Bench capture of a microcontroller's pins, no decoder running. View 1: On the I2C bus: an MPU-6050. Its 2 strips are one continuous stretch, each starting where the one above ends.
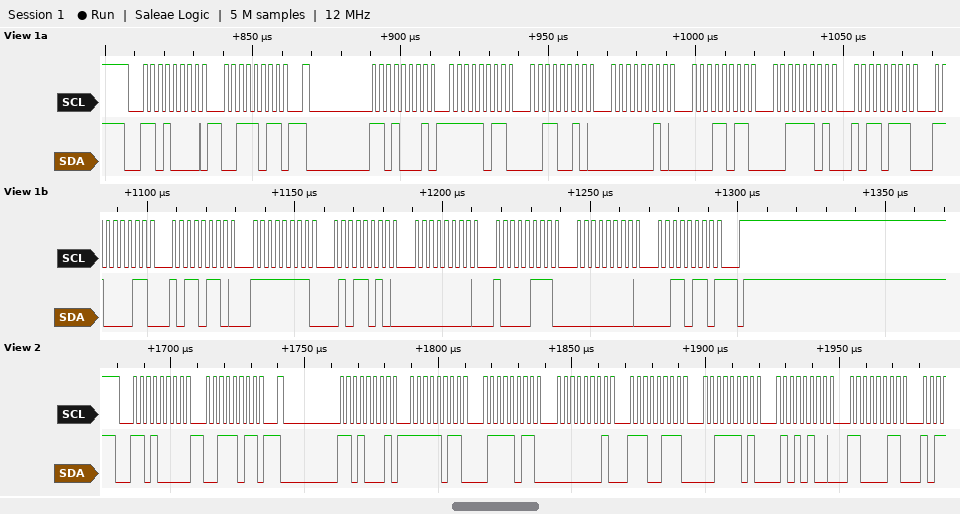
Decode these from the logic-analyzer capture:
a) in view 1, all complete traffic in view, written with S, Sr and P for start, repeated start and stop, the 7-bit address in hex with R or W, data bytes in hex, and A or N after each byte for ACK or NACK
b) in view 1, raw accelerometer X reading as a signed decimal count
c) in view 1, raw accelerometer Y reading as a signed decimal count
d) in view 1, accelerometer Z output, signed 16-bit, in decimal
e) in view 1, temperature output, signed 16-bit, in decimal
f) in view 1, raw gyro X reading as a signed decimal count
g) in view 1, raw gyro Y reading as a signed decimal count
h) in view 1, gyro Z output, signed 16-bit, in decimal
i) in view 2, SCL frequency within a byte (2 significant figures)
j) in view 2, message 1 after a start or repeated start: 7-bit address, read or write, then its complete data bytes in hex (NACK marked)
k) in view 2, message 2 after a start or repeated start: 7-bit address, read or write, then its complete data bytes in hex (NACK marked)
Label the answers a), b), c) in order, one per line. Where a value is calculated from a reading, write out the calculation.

a) S 68W A 3B A Sr 68R A FB A 32 A 02 A 1B A 3D A B7 A C3 A B6 A FF A 5A A 00 A 87 A 00 A 36 N P
b) 0xFB32 = -1230
c) 0x021B = 539
d) 0x3DB7 = 15799
e) 0xC3B6 = -15434
f) 0xFF5A = -166
g) 0x0087 = 135
h) 0x0036 = 54
i) 400 kHz
j) 0x68 write: 3B
k) 0x68 read: FB 7B 01 E7 3D 54 C3
